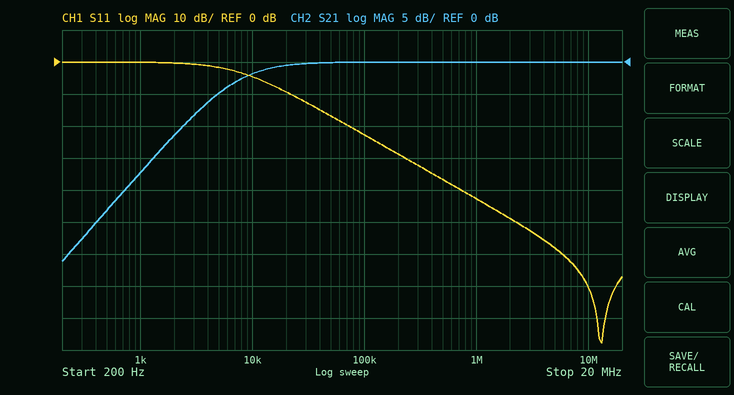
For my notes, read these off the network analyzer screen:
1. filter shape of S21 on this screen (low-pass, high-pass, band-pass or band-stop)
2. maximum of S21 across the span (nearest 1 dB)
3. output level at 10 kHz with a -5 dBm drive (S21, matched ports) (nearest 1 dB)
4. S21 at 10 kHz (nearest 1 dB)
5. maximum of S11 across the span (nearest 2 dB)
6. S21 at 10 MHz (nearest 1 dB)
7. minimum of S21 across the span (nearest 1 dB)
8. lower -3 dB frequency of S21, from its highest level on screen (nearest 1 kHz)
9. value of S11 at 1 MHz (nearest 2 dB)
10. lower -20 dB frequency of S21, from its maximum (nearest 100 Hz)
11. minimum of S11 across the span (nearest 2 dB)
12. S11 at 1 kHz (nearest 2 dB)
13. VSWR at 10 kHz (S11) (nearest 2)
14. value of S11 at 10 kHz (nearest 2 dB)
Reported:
high-pass
0 dB
-7 dBm
-2 dB
0 dB
0 dB
-31 dB
7 kHz
-42 dB
700 Hz
-88 dB
0 dB
4
-4 dB
